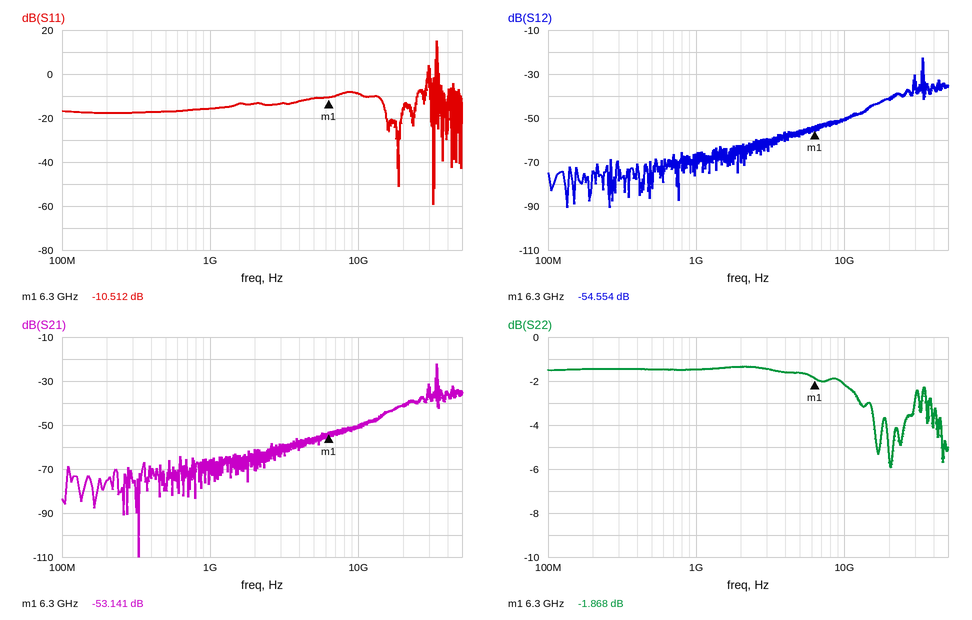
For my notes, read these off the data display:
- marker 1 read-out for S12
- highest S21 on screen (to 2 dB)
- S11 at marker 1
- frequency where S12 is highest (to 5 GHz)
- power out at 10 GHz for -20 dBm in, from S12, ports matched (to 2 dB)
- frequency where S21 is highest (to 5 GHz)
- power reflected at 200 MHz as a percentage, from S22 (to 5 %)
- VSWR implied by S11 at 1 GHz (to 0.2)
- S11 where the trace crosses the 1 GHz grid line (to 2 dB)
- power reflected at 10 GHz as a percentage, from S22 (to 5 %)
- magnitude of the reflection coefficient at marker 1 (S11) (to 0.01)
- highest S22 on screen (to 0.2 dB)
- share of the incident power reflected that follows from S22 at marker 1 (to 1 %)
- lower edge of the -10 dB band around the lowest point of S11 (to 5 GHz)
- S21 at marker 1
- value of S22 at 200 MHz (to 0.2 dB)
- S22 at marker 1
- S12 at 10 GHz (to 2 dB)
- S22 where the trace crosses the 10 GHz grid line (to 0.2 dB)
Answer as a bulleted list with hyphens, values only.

- -54.554 dB
- -22 dB
- -10.512 dB
- 35 GHz
- -70 dBm
- 35 GHz
- 70 %
- 1.4
- -16 dB
- 60 %
- 0.30
- -1.4 dB
- 65 %
- 30 GHz
- -53.141 dB
- -1.4 dB
- -1.868 dB
- -50 dB
- -2.2 dB
